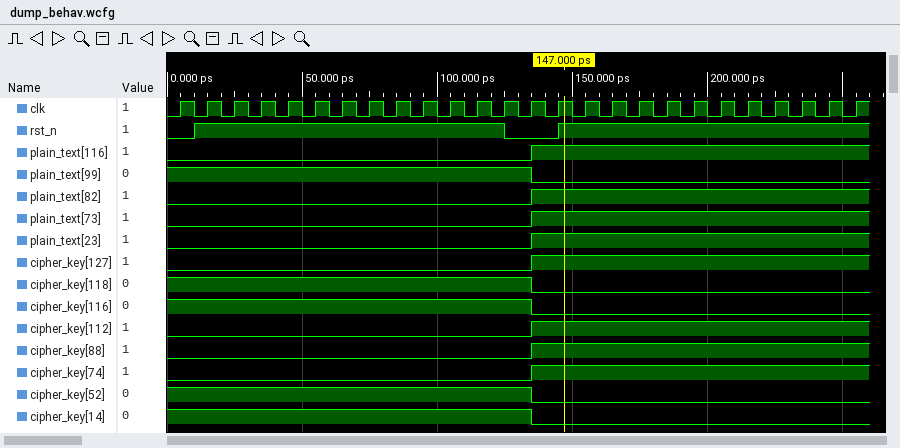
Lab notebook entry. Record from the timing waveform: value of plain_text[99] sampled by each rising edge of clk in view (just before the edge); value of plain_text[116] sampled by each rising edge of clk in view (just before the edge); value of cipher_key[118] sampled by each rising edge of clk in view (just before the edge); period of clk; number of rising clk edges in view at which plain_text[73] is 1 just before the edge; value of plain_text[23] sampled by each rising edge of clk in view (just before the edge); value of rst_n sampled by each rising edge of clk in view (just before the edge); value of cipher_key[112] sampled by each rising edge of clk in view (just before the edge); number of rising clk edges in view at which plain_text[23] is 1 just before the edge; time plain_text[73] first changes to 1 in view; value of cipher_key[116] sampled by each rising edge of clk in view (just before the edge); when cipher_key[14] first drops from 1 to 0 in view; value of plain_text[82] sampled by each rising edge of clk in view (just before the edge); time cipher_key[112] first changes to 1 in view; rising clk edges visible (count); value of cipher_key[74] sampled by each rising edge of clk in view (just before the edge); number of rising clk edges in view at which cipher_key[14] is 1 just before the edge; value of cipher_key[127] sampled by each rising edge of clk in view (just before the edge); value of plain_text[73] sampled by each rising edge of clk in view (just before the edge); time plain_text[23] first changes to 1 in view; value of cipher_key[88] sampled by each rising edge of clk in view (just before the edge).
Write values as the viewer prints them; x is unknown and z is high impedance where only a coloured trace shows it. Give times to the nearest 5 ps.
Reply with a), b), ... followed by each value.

a) 1 1 1 1 1 1 1 1 1 1 1 1 1 1 0 0 0 0 0 0 0 0 0 0 0 0
b) 0 0 0 0 0 0 0 0 0 0 0 0 0 0 1 1 1 1 1 1 1 1 1 1 1 1
c) 1 1 1 1 1 1 1 1 1 1 1 1 1 1 0 0 0 0 0 0 0 0 0 0 0 0
d) 10 ps
e) 12
f) 0 0 0 0 0 0 0 0 0 0 0 0 0 0 1 1 1 1 1 1 1 1 1 1 1 1
g) 0 1 1 1 1 1 1 1 1 1 1 1 1 0 0 1 1 1 1 1 1 1 1 1 1 1
h) 0 0 0 0 0 0 0 0 0 0 0 0 0 0 1 1 1 1 1 1 1 1 1 1 1 1
i) 12
j) 135 ps
k) 1 1 1 1 1 1 1 1 1 1 1 1 1 1 0 0 0 0 0 0 0 0 0 0 0 0
l) 135 ps
m) 0 0 0 0 0 0 0 0 0 0 0 0 0 0 1 1 1 1 1 1 1 1 1 1 1 1
n) 135 ps
o) 26
p) 0 0 0 0 0 0 0 0 0 0 0 0 0 0 1 1 1 1 1 1 1 1 1 1 1 1
q) 14
r) 0 0 0 0 0 0 0 0 0 0 0 0 0 0 1 1 1 1 1 1 1 1 1 1 1 1
s) 0 0 0 0 0 0 0 0 0 0 0 0 0 0 1 1 1 1 1 1 1 1 1 1 1 1
t) 135 ps
u) 0 0 0 0 0 0 0 0 0 0 0 0 0 0 1 1 1 1 1 1 1 1 1 1 1 1
